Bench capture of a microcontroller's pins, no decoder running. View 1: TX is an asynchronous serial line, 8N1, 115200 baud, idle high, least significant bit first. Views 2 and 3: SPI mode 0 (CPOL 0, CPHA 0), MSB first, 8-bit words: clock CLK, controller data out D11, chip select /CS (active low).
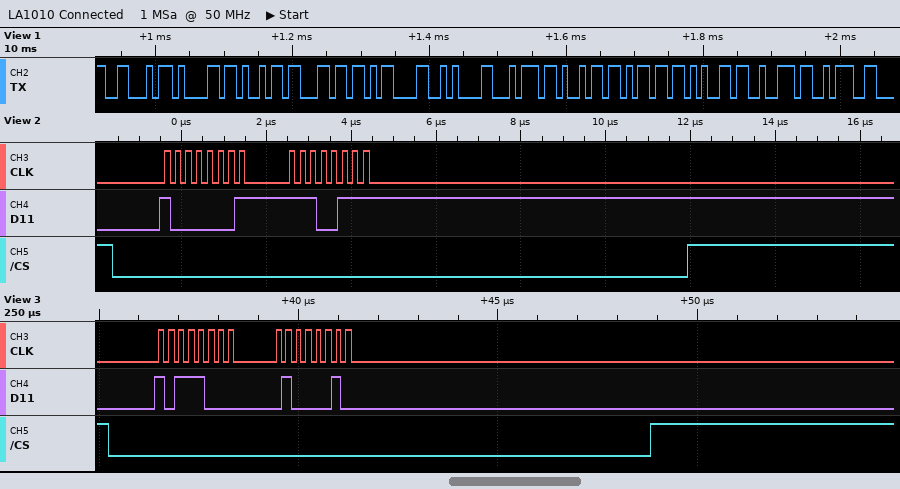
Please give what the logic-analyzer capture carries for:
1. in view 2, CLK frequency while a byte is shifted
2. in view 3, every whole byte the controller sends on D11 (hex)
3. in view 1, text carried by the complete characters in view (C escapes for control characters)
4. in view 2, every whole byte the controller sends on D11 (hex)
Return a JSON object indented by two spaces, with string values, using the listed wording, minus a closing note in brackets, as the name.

{
  "in view 2, CLK frequency while a byte is shifted": "4 MHz",
  "in view 3, every whole byte the controller sends on D11": "0xB8 0x42",
  "in view 1, text carried by the complete characters in view": "\"Fail\\r\\ntimer:\"",
  "in view 2, every whole byte the controller sends on D11": "81 E7"
}
